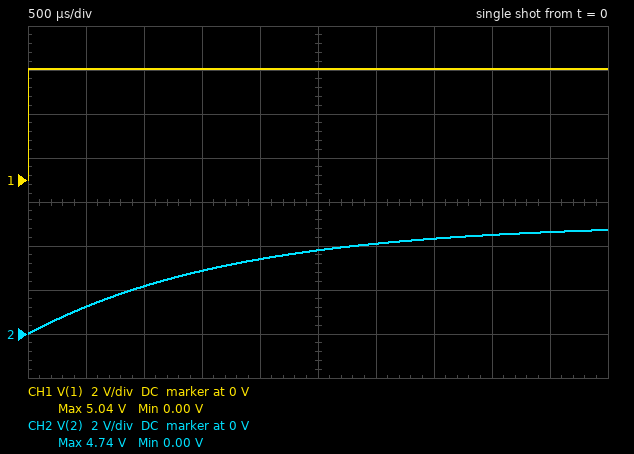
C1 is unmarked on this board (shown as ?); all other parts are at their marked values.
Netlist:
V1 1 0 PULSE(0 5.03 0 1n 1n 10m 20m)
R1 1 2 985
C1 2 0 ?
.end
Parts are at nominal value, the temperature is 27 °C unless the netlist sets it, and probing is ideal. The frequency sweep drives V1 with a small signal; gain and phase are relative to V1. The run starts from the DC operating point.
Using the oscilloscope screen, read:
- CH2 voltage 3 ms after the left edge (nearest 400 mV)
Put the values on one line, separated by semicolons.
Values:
4.0 V
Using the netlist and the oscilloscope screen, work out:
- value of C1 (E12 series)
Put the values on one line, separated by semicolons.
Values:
1.8 µF
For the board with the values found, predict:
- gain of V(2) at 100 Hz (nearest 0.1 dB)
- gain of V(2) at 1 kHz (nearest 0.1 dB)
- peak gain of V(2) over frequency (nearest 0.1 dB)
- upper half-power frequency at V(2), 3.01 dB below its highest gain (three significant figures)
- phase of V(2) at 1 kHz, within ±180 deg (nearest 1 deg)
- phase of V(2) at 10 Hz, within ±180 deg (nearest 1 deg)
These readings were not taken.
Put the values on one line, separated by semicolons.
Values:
-3.5 dB; -21.0 dB; 0 dB; 89.8 Hz; -85 deg; -6 deg
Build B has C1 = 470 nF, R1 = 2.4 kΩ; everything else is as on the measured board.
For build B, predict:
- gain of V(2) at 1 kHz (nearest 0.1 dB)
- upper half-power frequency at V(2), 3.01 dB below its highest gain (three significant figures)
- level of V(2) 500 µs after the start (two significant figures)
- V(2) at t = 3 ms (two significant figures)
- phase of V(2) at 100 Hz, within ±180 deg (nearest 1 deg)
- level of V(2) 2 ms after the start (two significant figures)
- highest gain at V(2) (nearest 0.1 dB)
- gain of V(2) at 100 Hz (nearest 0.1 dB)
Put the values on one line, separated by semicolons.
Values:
-17.1 dB; 141 Hz; 1.8 V; 4.7 V; -35 deg; 4.2 V; 0 dB; -1.8 dB
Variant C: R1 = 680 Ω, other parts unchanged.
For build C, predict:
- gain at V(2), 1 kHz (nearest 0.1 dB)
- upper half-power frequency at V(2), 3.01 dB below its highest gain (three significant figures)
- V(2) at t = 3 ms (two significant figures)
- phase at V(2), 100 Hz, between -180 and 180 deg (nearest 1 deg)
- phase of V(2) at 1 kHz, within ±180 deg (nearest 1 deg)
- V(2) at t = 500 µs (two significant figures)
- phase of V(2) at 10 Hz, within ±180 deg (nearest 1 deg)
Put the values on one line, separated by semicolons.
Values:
-17.8 dB; 130 Hz; 4.6 V; -38 deg; -83 deg; 1.7 V; -4 deg
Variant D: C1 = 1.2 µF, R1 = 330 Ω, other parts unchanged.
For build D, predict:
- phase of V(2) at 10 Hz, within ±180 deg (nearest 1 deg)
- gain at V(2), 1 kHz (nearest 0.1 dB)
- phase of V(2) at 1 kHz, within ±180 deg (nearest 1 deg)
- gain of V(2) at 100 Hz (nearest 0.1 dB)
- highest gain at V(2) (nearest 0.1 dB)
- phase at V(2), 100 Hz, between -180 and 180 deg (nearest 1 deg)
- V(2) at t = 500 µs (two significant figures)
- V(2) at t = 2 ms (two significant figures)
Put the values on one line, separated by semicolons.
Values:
-1 deg; -8.6 dB; -68 deg; -0.3 dB; 0 dB; -14 deg; 3.6 V; 5.0 V
